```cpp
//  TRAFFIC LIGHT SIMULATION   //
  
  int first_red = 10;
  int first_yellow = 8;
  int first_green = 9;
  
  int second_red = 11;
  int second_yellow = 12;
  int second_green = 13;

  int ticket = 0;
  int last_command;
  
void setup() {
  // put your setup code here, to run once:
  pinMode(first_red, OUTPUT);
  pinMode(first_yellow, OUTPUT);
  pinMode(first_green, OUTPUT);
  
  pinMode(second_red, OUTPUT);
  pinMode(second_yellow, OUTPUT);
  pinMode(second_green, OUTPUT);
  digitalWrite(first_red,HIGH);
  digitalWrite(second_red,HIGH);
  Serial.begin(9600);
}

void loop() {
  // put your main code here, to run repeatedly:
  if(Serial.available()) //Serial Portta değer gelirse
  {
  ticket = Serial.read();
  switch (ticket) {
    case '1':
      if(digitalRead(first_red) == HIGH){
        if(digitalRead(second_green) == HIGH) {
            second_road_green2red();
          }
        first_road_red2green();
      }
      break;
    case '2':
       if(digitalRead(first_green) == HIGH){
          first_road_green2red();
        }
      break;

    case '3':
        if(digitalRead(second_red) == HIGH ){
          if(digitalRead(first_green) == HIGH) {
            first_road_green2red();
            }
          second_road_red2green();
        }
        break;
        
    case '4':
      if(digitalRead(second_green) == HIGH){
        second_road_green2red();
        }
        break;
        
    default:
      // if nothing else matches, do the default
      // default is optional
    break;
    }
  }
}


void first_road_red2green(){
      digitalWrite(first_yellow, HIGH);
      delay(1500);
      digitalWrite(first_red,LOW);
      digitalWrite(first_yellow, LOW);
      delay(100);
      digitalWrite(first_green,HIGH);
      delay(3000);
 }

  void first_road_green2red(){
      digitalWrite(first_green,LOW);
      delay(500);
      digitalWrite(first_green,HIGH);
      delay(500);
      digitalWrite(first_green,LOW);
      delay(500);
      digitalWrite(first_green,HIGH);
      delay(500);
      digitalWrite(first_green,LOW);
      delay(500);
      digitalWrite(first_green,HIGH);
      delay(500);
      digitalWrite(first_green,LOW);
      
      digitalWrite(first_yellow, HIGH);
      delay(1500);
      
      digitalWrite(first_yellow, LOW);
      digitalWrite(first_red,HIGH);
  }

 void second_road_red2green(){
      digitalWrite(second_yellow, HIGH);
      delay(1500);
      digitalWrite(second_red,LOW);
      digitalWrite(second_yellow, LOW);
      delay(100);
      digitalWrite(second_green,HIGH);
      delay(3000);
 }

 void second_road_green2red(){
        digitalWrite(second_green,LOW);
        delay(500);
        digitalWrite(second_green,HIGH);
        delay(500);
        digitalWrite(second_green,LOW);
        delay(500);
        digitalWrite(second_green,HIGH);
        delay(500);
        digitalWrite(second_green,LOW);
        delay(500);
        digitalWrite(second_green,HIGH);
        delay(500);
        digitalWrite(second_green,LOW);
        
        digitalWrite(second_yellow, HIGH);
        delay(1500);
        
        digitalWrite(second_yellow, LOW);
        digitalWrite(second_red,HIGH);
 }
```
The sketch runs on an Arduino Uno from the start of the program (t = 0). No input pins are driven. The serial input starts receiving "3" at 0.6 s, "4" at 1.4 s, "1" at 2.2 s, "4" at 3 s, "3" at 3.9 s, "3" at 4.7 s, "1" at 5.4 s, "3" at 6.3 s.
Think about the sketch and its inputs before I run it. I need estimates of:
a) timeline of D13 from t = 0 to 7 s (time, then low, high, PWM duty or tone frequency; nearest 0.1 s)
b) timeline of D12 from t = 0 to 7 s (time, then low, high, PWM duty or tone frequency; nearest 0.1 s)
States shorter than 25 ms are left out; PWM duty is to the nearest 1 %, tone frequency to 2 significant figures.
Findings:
0 s low; 2.2 s high; 5.2 s low; 5.7 s high; 6.2 s low; 6.7 s high
0 s low; 0.6 s high; 2.1 s low
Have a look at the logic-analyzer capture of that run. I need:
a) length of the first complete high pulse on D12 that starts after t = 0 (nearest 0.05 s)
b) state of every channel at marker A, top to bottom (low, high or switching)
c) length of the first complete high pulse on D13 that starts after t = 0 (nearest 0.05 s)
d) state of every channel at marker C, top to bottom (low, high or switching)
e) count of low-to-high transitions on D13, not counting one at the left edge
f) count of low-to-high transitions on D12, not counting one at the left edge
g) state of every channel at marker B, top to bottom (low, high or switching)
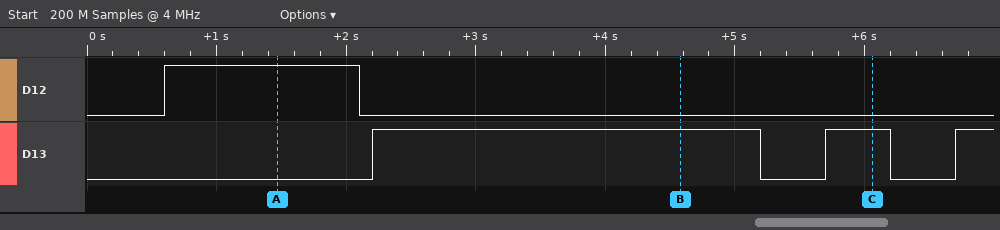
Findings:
1.50 s
D12 high, D13 low
3.00 s
D12 low, D13 high
3
1
D12 low, D13 high
